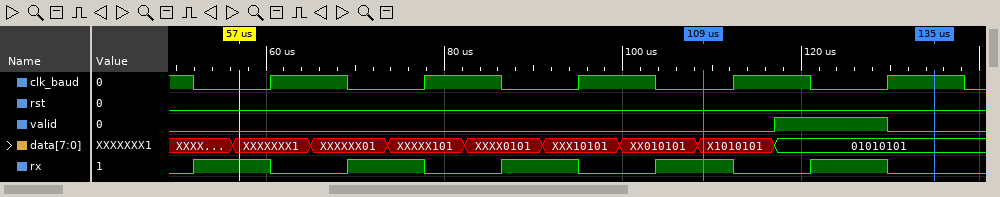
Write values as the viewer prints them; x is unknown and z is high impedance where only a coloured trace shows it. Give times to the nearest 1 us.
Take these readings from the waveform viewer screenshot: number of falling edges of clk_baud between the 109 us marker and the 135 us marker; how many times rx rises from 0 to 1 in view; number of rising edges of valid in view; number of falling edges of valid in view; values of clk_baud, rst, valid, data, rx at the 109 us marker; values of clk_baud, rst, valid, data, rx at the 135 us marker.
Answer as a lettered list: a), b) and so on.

a) 1
b) 5
c) 1
d) 1
e) clk_baud=0, rst=0, valid=0, data=X1010101, rx=1
f) clk_baud=1, rst=0, valid=0, data=01010101, rx=0
